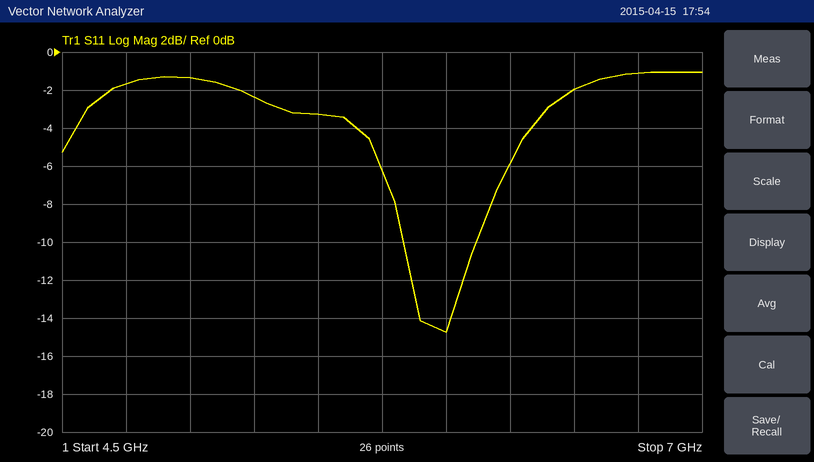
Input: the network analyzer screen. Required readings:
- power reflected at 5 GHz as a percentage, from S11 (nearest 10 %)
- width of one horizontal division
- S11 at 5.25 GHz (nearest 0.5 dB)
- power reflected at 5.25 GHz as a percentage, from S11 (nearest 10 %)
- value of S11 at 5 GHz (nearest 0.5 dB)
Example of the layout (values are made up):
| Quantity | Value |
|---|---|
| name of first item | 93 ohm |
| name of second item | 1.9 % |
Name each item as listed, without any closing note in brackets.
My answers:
| Quantity | Value |
|---|---|
| power reflected at 5 GHz as a percentage, from S11 | 70 % |
| width of one horizontal division | 250 MHz |
| S11 at 5.25 GHz | -2.5 dB |
| power reflected at 5.25 GHz as a percentage, from S11 | 60 % |
| value of S11 at 5 GHz | -1.5 dB |
